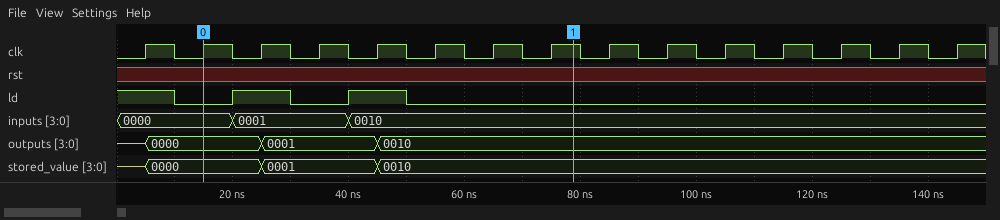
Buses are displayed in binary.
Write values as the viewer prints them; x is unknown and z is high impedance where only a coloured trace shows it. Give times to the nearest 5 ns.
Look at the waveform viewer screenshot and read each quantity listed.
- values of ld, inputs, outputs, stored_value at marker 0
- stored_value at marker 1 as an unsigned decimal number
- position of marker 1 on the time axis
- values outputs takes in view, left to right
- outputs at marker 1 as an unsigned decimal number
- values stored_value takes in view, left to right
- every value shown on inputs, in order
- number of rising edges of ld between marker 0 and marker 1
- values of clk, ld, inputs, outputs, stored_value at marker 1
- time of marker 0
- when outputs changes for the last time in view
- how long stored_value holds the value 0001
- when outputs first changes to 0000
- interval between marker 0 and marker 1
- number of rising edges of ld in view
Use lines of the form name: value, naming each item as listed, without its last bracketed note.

values of ld, inputs, outputs, stored_value at marker 0: ld=0, inputs=0000, outputs=0000, stored_value=0000
stored_value at marker 1 as an unsigned decimal number: 2
position of marker 1 on the time axis: 80 ns
values outputs takes in view, left to right: z, 0000, 0001, 0010
outputs at marker 1 as an unsigned decimal number: 2
values stored_value takes in view, left to right: z, 0000, 0001, 0010
every value shown on inputs, in order: 0000, 0001, 0010
number of rising edges of ld between marker 0 and marker 1: 2
values of clk, ld, inputs, outputs, stored_value at marker 1: clk=1, ld=0, inputs=0010, outputs=0010, stored_value=0010
time of marker 0: 15 ns
when outputs changes for the last time in view: 45 ns
how long stored_value holds the value 0001: 20 ns
when outputs first changes to 0000: 5 ns
interval between marker 0 and marker 1: 65 ns
number of rising edges of ld in view: 2
